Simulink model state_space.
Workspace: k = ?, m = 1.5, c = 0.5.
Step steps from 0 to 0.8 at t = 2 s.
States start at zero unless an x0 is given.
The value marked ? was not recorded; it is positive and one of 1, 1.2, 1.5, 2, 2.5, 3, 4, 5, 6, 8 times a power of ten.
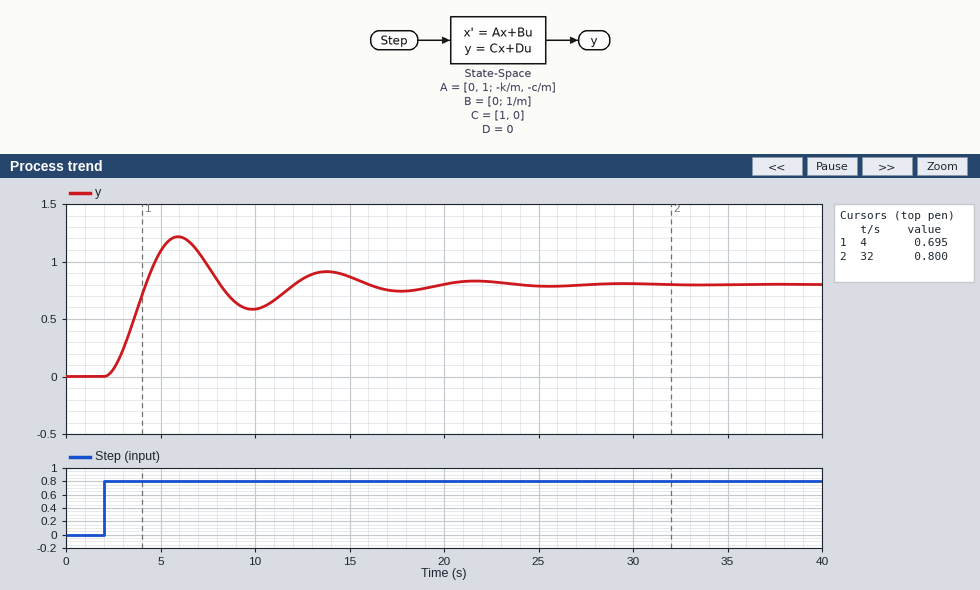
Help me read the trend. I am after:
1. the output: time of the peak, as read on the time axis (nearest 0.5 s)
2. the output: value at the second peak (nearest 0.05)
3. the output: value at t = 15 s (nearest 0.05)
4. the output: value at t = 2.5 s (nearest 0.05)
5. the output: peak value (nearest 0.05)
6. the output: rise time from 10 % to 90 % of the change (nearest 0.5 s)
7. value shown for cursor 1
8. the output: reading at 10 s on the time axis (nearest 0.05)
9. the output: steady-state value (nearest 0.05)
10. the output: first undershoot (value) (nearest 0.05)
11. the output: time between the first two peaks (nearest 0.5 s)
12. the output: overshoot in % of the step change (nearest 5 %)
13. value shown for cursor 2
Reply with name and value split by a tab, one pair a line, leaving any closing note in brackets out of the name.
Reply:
the output: time of the peak, as read on the time axis	6.0 s
the output: value at the second peak	0.90
the output: value at t = 15 s	0.85
the output: value at t = 2.5 s	0.05
the output: peak value	1.20
the output: rise time from 10 % to 90 % of the change	1.5 s
value shown for cursor 1	0.695
the output: reading at 10 s on the time axis	0.60
the output: steady-state value	0.80
the output: first undershoot (value)	0.60
the output: time between the first two peaks	8.0 s
the output: overshoot in % of the step change	50 %
value shown for cursor 2	0.800
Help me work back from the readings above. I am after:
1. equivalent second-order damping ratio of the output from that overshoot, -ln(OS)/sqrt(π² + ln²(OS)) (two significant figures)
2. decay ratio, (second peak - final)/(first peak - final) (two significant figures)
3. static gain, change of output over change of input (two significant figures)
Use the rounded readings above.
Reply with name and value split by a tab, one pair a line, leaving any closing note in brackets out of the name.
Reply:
equivalent second-order damping ratio of the output from that overshoot, -ln(OS)/sqrt(π² + ln²(OS))	0.22
decay ratio, (second peak - final)/(first peak - final)	0.25
static gain, change of output over change of input	1.0
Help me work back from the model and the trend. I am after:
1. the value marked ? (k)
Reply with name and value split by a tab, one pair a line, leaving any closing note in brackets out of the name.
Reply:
the value marked ?	1
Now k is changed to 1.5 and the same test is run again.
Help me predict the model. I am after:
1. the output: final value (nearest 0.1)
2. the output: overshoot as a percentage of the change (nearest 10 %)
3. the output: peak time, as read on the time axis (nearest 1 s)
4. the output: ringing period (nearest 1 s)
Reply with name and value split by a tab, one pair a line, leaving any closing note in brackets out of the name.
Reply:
the output: final value	0.5
the output: overshoot as a percentage of the change	60 %
the output: peak time, as read on the time axis	5 s
the output: ringing period	6 s
